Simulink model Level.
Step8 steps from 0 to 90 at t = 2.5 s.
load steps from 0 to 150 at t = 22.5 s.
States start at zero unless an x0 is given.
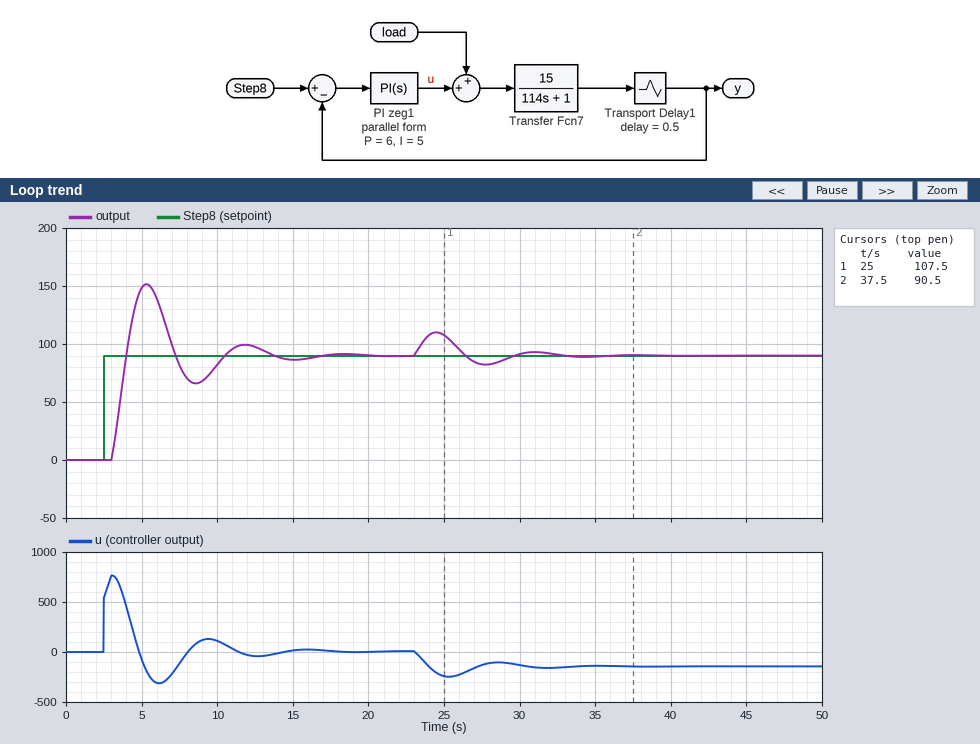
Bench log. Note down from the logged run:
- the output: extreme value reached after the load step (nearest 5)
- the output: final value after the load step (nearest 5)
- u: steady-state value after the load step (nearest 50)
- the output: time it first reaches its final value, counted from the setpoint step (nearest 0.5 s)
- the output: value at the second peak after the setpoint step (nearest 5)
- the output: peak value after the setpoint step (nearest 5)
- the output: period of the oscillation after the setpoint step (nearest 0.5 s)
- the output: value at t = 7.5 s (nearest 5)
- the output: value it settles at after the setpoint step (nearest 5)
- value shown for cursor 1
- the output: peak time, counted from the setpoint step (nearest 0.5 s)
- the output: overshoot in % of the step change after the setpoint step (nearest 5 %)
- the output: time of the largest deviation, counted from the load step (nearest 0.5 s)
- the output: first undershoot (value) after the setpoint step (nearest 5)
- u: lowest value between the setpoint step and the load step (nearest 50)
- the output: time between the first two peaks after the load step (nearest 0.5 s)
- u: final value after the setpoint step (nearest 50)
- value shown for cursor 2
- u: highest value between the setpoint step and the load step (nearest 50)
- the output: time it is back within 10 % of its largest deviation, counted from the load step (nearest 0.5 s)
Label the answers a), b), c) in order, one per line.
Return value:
a) 110
b) 90
c) -150
d) 1.5 s
e) 100
f) 150
g) 6.5 s
h) 80
i) 90
j) 107.5
k) 3.0 s
l) 70 %
m) 2.0 s
n) 65
o) -300
p) 6.5 s
q) 0
r) 90.5
s) 750
t) 9.5 s
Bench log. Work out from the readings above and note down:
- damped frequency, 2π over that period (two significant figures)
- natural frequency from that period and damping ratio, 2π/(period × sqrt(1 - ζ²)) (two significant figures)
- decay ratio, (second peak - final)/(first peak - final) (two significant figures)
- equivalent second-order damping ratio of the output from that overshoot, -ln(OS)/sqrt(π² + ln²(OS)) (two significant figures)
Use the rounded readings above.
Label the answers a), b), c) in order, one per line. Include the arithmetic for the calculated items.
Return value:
a) 2π / 6.5 = 0.97 rad/s
b) 2π / (6.5 × sqrt(1 - 0.11²)) = 0.97 rad/s
c) (100 - 90) / (150 - 90) = 0.17
d) ln(0.7) = -0.357; 0.357 / sqrt(9.870 + 0.127) = 0.11
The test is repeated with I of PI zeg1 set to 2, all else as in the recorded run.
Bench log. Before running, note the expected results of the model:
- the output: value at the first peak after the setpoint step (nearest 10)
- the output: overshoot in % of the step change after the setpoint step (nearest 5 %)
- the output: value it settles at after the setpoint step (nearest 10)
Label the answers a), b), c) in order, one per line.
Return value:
a) 120
b) 30 %
c) 90
